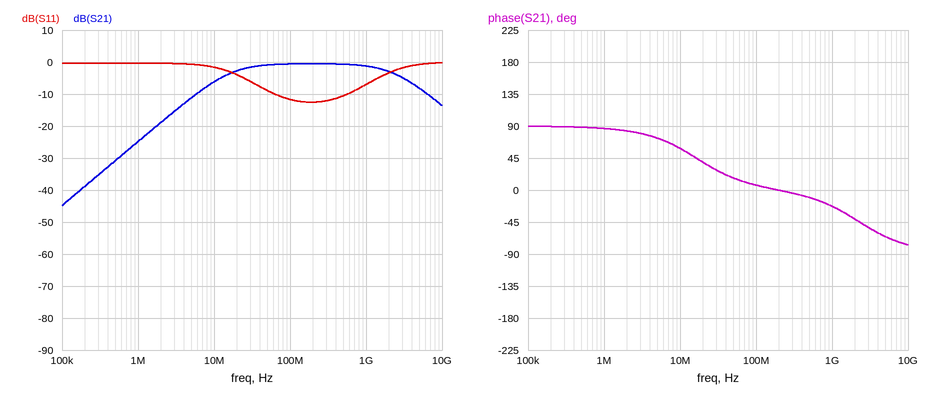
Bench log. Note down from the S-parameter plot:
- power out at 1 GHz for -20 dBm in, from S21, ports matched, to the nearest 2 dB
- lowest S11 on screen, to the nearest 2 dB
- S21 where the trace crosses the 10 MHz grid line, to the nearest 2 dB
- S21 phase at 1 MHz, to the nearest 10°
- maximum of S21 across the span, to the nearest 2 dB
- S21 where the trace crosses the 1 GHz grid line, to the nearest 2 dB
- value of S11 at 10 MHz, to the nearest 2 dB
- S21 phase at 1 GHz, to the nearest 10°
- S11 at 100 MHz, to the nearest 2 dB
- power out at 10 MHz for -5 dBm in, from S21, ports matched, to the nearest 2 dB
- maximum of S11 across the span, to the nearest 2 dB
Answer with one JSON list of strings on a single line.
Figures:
["-22 dBm", "-12 dB", "-6 dB", "90°", "0 dB", "-2 dB", "-2 dB", "-20°", "-12 dB", "-12 dBm", "0 dB"]
